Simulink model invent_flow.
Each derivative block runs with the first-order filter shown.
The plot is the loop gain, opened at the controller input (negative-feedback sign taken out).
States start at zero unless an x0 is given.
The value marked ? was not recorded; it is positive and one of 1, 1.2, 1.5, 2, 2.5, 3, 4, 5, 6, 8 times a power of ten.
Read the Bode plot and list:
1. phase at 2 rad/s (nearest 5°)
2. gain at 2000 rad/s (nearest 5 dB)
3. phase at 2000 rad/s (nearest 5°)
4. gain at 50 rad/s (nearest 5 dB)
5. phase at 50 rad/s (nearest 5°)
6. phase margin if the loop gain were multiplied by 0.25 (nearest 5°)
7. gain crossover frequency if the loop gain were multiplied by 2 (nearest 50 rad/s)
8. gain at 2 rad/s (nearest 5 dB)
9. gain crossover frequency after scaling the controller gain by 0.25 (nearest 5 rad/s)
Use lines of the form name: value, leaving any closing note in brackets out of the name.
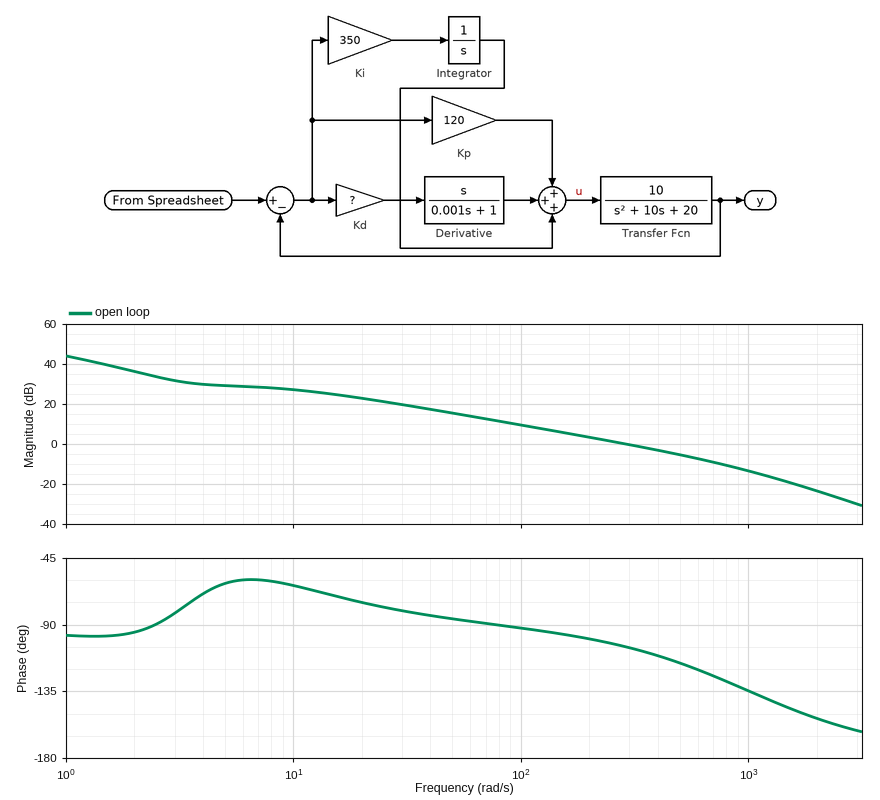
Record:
phase at 2 rad/s: -95°
gain at 2000 rad/s: -25 dB
phase at 2000 rad/s: -155°
gain at 50 rad/s: 15 dB
phase at 50 rad/s: -85°
phase margin if the loop gain were multiplied by 0.25: 90°
gain crossover frequency if the loop gain were multiplied by 2: 550 rad/s
gain at 2 rad/s: 35 dB
gain crossover frequency after scaling the controller gain by 0.25: 75 rad/s
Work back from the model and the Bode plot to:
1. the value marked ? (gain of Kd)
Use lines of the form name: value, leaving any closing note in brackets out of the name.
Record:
the value marked ?: 30
